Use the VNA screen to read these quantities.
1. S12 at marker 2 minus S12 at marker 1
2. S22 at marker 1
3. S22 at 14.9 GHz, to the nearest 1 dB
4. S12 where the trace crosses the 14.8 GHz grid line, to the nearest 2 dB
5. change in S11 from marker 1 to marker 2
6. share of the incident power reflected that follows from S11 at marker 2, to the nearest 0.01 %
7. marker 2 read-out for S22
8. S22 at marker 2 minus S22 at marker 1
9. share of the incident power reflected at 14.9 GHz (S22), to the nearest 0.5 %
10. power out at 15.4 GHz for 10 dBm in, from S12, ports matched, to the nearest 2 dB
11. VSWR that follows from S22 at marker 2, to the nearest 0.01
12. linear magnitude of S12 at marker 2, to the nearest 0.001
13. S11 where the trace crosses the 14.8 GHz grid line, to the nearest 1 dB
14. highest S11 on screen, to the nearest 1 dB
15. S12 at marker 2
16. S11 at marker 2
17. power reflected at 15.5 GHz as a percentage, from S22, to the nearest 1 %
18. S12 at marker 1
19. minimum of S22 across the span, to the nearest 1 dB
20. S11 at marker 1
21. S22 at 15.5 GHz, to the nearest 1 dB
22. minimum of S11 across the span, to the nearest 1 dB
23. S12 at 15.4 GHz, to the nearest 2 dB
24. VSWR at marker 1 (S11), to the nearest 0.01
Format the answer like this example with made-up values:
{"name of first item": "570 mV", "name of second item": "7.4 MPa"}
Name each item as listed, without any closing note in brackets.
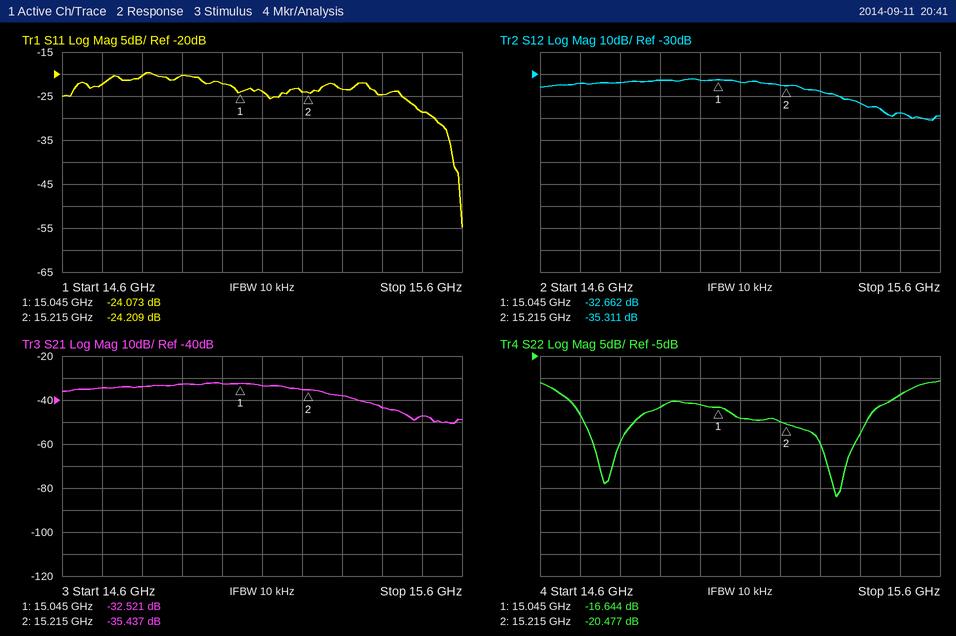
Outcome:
{"S12 at marker 2 minus S12 at marker 1": "-2.649 dB", "S22 at marker 1": "-16.644 dB", "S22 at 14.9 GHz, to the nearest 1 dB": "-17 dB", "S12 where the trace crosses the 14.8 GHz grid line, to the nearest 2 dB": "-34 dB", "change in S11 from marker 1 to marker 2": "-0.136 dB", "share of the incident power reflected that follows from S11 at marker 2, to the nearest 0.01 %": "0.38 %", "marker 2 read-out for S22": "-20.477 dB", "S22 at marker 2 minus S22 at marker 1": "-3.833 dB", "share of the incident power reflected at 14.9 GHz (S22), to the nearest 0.5 %": "2.0 %", "power out at 15.4 GHz for 10 dBm in, from S12, ports matched, to the nearest 2 dB": "-34 dBm", "VSWR that follows from S22 at marker 2, to the nearest 0.01": "1.21", "linear magnitude of S12 at marker 2, to the nearest 0.001": "0.017", "S11 where the trace crosses the 14.8 GHz grid line, to the nearest 1 dB": "-20 dB", "highest S11 on screen, to the nearest 1 dB": "-20 dB", "S12 at marker 2": "-35.311 dB", "S11 at marker 2": "-24.209 dB", "power reflected at 15.5 GHz as a percentage, from S22, to the nearest 1 %": "4 %", "S12 at marker 1": "-32.662 dB", "minimum of S22 across the span, to the nearest 1 dB": "-37 dB", "S11 at marker 1": "-24.073 dB", "S22 at 15.5 GHz, to the nearest 1 dB": "-14 dB", "minimum of S11 across the span, to the nearest 1 dB": "-55 dB", "S12 at 15.4 GHz, to the nearest 2 dB": "-44 dB", "VSWR at marker 1 (S11), to the nearest 0.01": "1.13"}
